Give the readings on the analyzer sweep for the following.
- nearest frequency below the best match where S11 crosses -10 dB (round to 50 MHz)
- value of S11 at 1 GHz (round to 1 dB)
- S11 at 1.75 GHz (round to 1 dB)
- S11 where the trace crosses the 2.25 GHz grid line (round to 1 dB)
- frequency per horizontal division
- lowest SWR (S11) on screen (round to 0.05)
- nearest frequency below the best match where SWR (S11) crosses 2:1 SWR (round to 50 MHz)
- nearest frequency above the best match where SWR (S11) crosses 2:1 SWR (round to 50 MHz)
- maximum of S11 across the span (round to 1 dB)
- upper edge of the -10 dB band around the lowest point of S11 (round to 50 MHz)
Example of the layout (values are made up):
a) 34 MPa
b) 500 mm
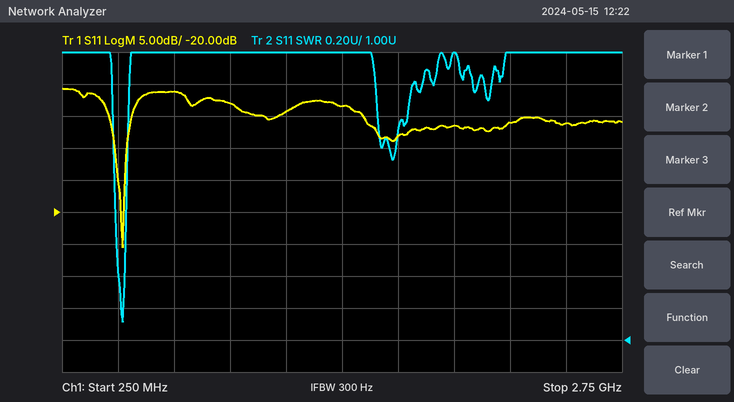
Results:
a) 500 MHz
b) -3 dB
c) -8 dB
d) -6 dB
e) 250 MHz
f) 1.10
g) 500 MHz
h) 550 MHz
i) -1 dB
j) 550 MHz
